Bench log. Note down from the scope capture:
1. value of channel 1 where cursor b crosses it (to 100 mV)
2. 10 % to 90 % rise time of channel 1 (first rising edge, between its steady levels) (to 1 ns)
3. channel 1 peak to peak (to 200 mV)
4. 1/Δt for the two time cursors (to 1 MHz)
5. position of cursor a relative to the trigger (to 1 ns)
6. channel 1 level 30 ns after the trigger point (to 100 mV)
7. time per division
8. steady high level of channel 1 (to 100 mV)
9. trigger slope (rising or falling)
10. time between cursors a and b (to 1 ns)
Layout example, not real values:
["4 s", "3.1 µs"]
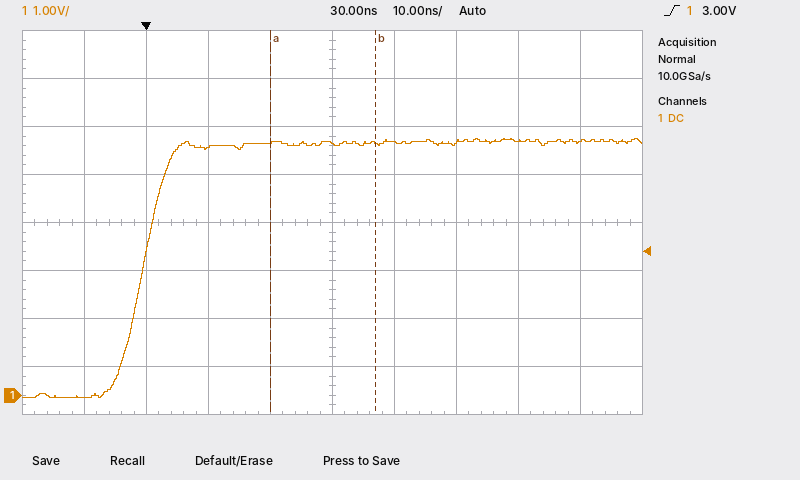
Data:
["5.2 V", "8 ns", "5.4 V", "59 MHz", "+20 ns", "5.2 V", "10 ns", "5.3 V", "rising", "17 ns"]
